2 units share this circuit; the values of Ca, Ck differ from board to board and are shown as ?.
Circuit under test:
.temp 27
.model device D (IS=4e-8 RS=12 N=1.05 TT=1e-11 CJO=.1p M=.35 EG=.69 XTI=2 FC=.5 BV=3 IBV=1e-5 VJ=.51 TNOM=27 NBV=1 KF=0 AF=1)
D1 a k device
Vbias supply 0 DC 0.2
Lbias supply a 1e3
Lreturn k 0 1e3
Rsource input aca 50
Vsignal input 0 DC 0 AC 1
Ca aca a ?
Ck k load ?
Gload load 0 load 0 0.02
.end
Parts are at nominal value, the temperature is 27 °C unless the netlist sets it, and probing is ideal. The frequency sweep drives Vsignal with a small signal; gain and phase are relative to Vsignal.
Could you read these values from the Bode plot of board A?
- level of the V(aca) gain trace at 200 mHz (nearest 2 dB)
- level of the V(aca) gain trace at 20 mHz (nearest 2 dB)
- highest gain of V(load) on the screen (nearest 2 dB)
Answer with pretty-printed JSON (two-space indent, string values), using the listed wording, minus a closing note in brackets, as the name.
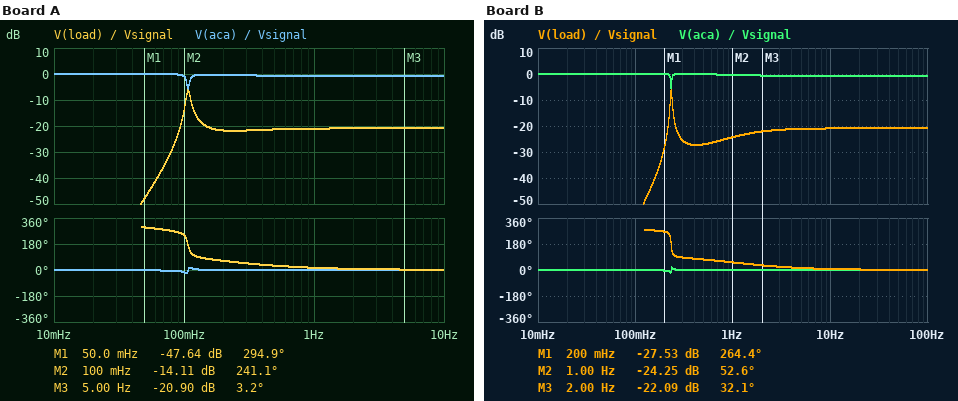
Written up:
{
  "level of the V(aca) gain trace at 200 mHz": "0 dB",
  "level of the V(aca) gain trace at 20 mHz": "0 dB",
  "highest gain of V(load) on the screen": "-6 dB"
}
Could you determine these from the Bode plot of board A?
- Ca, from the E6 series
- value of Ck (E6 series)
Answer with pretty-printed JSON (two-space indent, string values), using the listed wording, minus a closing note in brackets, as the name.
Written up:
{
  "Ca, from the E6 series": "2.2 mF",
  "value of Ck": "2.2 mF"
}
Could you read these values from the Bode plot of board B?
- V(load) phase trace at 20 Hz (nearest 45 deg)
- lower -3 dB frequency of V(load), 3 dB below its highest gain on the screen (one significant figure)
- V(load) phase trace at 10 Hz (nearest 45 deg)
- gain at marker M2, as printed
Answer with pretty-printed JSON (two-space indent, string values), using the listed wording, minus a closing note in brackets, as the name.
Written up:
{
  "V(load) phase trace at 20 Hz": "0 deg",
  "lower -3 dB frequency of V(load), 3 dB below its highest gain on the screen": "200 mHz",
  "V(load) phase trace at 10 Hz": "0 deg",
  "gain at marker M2, as printed": "-24.25 dB"
}
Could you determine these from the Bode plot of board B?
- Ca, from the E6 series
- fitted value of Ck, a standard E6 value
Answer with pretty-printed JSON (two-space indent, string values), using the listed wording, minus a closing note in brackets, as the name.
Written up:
{
  "Ca, from the E6 series": "470 µF",
  "fitted value of Ck, a standard E6 value": "470 µF"
}
